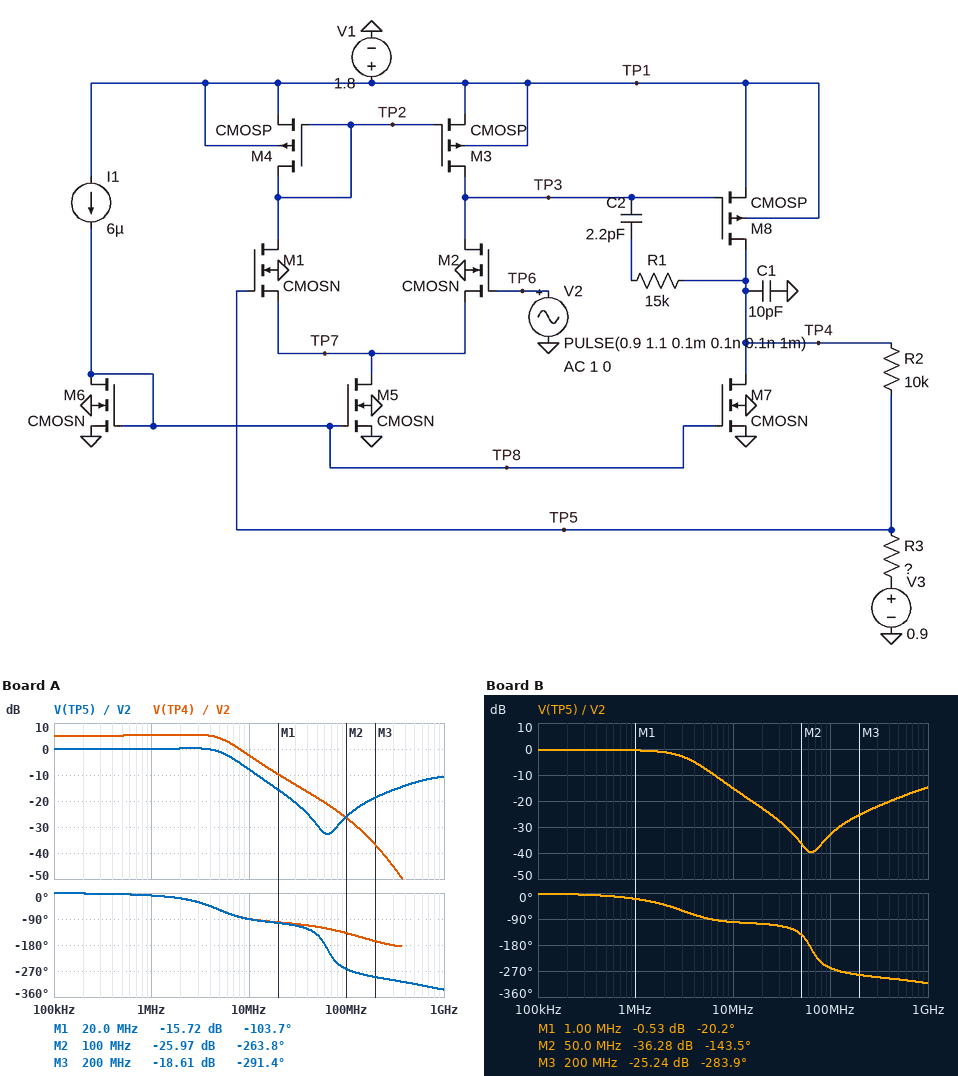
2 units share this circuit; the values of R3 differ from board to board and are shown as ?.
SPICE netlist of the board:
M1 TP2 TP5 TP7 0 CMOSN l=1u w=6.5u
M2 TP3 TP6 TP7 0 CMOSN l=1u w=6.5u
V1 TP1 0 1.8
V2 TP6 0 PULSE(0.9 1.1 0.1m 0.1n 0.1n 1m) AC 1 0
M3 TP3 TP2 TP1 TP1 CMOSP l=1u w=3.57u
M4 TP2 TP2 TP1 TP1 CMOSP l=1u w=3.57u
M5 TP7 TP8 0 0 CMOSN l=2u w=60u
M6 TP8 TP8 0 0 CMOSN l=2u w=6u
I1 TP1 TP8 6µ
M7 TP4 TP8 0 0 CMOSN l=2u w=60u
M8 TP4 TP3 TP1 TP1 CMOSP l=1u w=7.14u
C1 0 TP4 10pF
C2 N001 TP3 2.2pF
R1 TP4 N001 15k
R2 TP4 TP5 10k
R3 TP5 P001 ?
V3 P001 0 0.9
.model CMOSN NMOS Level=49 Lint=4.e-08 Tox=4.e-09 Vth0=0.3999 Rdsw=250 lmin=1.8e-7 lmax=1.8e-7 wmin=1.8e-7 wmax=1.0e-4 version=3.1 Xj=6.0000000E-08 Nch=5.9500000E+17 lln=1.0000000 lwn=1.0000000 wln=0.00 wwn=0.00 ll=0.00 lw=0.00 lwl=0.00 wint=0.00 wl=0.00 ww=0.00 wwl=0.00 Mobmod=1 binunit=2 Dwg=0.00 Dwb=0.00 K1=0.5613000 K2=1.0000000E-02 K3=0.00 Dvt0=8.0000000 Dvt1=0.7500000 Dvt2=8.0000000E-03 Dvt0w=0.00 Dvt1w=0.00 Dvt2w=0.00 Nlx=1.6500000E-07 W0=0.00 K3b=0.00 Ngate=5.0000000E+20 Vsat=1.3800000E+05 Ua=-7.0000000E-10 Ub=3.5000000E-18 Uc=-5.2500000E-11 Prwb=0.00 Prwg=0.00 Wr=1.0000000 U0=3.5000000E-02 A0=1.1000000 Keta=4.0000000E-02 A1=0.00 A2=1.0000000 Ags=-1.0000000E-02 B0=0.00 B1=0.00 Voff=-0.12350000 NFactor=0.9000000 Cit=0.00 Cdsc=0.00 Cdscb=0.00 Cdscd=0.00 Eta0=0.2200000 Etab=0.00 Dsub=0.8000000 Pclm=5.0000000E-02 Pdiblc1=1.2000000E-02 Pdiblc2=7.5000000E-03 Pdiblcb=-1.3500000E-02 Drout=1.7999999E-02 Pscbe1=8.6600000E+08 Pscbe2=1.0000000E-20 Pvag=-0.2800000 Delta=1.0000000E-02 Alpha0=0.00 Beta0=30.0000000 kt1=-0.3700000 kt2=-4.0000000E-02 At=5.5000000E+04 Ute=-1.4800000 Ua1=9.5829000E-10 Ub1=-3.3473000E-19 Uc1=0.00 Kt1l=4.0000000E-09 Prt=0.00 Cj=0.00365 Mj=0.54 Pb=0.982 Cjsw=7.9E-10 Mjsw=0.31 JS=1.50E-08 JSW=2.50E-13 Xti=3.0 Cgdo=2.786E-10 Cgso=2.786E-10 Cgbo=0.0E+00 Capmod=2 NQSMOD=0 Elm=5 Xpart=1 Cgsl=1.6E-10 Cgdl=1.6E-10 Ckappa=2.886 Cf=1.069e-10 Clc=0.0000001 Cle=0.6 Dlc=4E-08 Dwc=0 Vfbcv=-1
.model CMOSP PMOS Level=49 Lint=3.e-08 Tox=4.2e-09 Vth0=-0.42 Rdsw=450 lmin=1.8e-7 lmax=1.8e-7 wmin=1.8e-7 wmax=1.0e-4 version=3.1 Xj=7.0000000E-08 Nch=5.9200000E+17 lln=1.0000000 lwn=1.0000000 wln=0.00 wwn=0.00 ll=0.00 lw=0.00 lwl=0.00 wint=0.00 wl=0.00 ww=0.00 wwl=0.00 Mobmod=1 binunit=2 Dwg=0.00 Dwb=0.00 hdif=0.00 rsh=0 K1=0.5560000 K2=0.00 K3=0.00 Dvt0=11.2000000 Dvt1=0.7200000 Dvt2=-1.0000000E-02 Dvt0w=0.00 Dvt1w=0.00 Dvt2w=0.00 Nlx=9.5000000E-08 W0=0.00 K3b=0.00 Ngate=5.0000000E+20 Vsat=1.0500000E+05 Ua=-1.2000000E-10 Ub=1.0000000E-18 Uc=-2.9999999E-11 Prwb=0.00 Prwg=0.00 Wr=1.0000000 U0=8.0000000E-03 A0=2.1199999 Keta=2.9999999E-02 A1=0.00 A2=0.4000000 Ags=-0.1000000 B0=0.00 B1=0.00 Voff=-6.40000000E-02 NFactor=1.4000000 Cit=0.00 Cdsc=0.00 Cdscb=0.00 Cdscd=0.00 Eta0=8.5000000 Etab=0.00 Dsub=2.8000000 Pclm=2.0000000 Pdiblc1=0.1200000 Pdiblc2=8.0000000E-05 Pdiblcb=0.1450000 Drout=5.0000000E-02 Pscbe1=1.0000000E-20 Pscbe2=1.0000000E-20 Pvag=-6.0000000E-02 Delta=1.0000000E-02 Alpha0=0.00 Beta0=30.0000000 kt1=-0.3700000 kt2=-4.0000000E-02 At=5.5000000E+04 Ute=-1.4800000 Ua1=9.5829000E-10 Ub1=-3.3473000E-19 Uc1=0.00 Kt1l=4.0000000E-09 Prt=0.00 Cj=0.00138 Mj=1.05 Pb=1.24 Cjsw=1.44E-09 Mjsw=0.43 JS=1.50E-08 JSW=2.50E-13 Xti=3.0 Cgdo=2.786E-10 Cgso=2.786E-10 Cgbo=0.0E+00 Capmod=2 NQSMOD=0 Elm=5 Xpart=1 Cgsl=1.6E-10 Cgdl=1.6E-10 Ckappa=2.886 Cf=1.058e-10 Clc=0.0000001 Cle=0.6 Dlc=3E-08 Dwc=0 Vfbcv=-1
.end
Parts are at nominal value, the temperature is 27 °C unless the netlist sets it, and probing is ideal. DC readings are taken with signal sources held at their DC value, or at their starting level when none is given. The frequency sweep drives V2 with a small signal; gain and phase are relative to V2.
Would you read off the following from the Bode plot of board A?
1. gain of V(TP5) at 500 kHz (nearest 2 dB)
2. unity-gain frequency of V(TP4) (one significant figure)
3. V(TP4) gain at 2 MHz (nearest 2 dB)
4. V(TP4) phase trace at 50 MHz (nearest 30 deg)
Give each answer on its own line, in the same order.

0 dB
8 MHz
6 dB
-120 deg
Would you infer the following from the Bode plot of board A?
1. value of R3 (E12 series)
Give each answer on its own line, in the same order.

12 kΩ
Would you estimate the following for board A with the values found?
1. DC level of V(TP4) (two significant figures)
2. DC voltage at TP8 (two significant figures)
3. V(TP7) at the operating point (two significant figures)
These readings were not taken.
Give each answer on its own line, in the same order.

900 mV
520 mV
220 mV
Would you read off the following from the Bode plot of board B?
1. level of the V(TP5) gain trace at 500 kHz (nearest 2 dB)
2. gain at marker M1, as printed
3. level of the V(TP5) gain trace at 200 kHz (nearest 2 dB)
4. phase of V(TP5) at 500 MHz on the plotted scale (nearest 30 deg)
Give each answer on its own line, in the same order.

0 dB
-0.53 dB
0 dB
-300 deg
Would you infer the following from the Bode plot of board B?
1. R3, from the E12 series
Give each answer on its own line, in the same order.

3.3 kΩ
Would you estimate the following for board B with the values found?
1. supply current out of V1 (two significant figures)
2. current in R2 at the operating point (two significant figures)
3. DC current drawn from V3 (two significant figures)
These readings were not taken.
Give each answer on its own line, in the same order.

130 µA
140 nA
140 nA
